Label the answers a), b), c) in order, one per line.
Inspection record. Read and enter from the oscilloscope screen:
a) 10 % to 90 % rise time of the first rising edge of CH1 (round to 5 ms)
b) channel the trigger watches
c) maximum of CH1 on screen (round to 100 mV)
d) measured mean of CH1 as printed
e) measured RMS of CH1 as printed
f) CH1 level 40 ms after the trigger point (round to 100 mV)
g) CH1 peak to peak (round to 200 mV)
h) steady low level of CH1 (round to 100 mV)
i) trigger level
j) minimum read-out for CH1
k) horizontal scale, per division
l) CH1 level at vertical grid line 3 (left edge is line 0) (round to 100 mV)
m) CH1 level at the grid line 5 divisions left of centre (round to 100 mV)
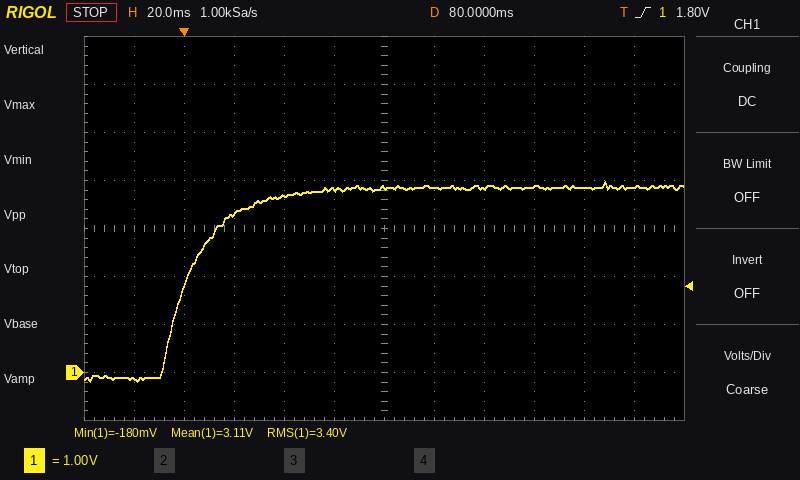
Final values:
a) 35 ms
b) CH1
c) 4.0 V
d) 3.11 V
e) 3.40 V
f) 3.7 V
g) 4.2 V
h) -100 mV
i) 1.80 V
j) -180 mV
k) 20 ms
l) 3.3 V
m) -100 mV
